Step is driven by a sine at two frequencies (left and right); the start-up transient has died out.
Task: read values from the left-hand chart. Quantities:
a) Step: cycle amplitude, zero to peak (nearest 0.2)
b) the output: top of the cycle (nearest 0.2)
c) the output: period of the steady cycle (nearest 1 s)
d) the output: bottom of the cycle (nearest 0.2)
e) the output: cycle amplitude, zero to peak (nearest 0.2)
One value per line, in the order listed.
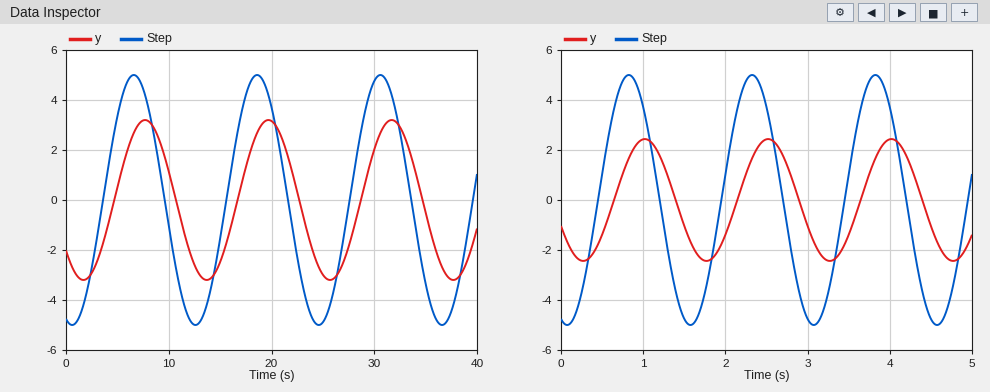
5.0
3.2
12 s
-3.2
3.2
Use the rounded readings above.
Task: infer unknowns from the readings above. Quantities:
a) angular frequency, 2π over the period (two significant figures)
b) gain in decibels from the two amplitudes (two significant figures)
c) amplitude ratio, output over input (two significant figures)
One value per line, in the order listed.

0.52 rad/s
-3.9 dB
0.64
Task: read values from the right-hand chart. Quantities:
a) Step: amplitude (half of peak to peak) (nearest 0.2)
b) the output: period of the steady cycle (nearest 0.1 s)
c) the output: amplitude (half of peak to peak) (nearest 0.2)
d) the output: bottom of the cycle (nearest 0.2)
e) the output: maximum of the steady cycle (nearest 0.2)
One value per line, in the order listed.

5.0
1.5 s
2.4
-2.4
2.4
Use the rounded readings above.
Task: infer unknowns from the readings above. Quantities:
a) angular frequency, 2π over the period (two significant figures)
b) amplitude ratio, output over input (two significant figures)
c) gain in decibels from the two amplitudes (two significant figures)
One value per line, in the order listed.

4.2 rad/s
0.48
-6.4 dB
